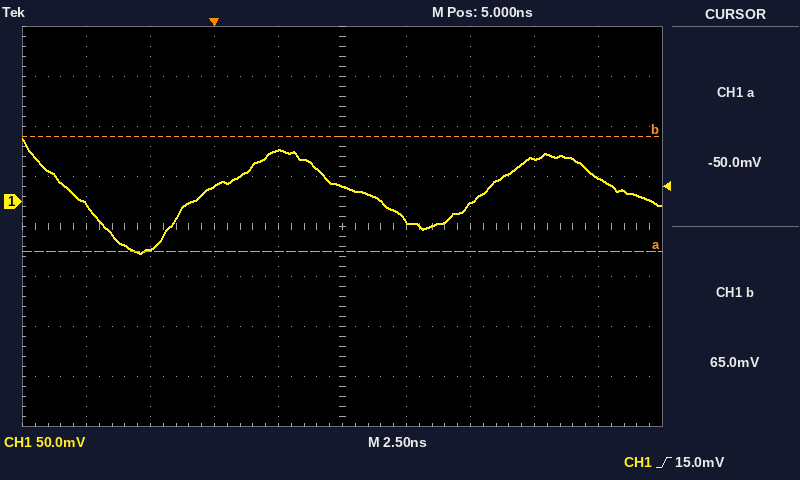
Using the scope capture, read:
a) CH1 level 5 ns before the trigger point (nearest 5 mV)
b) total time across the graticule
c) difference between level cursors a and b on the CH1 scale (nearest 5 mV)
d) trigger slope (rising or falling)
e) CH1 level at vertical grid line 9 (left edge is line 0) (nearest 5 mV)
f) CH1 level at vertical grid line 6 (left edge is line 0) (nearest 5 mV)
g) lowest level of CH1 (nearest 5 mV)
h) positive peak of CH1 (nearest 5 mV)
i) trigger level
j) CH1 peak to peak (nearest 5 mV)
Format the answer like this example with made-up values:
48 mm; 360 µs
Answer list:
-5 mV; 25 ns; 115 mV; rising; 25 mV; -20 mV; -50 mV; 65 mV; 15.0 mV; 115 mV
